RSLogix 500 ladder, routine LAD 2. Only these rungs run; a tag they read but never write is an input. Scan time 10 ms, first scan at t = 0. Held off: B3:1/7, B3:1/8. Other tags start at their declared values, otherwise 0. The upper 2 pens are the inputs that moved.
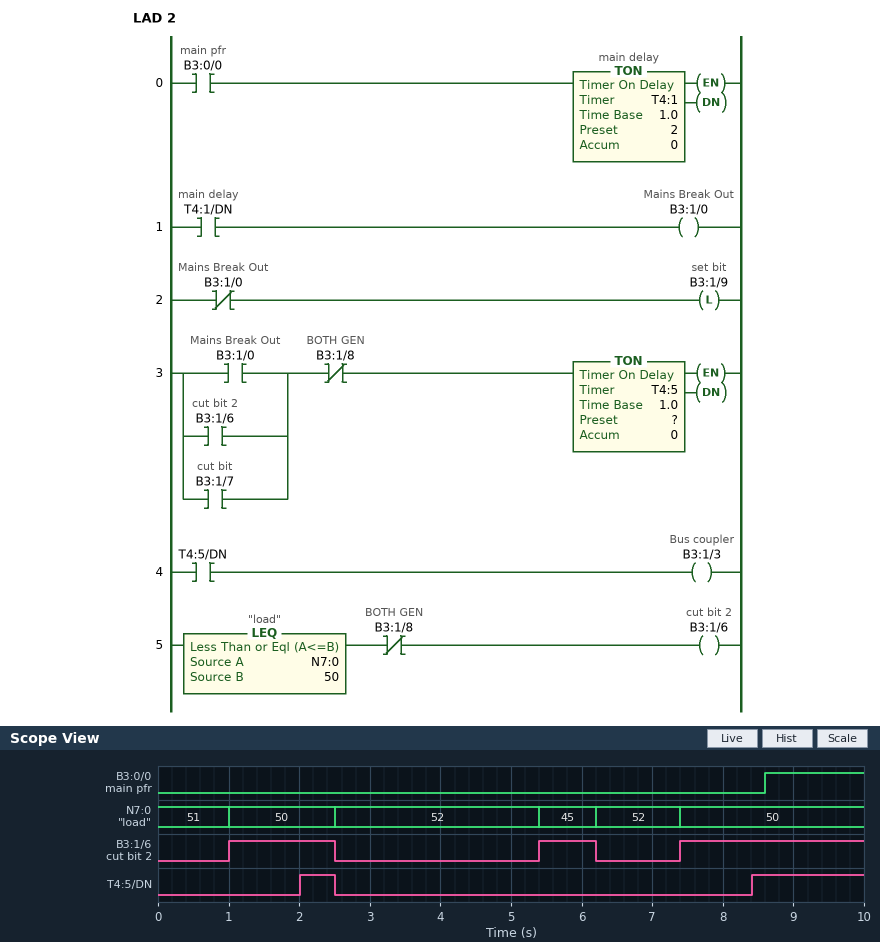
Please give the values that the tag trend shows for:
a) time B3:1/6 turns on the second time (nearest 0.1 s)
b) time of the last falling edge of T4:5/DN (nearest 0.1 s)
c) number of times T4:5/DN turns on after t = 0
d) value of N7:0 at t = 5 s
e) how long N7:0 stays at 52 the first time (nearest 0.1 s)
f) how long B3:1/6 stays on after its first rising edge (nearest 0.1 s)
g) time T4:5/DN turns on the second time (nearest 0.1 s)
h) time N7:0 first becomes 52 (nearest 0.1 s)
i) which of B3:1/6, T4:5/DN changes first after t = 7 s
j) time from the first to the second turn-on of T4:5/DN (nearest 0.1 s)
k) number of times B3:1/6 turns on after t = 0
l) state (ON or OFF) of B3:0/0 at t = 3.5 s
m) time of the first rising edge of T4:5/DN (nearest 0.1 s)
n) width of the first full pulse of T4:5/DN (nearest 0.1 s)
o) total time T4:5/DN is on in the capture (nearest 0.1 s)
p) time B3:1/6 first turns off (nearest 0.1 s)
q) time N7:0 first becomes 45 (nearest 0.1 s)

5.4 s
2.5 s
2
52
2.9 s
1.5 s
8.4 s
2.5 s
B3:1/6
6.4 s
3
OFF
2.0 s
0.5 s
2.1 s
2.5 s
5.4 s
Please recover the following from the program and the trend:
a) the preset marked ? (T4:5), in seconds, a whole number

1 s
